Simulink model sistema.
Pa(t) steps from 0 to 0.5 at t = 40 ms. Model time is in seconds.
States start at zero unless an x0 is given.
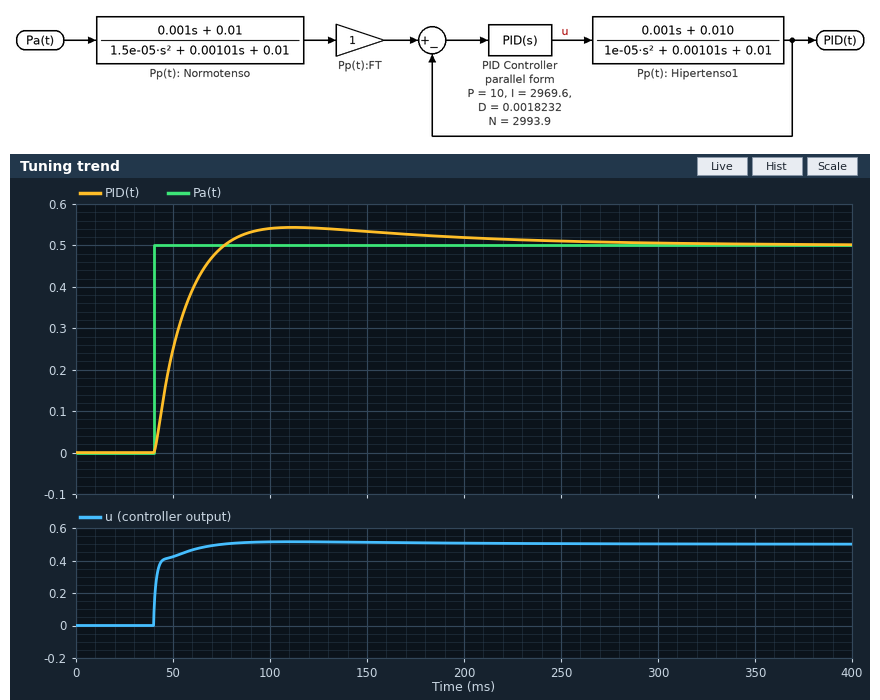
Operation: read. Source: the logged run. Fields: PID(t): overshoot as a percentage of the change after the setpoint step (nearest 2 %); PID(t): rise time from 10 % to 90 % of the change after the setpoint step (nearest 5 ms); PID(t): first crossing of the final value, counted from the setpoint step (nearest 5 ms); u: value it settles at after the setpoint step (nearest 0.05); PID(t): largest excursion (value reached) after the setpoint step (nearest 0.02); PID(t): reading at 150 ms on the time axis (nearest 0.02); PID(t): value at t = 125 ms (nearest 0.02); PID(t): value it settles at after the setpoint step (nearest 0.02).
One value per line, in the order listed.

8 %
25 ms
35 ms
0.50
0.54
0.54
0.54
0.50
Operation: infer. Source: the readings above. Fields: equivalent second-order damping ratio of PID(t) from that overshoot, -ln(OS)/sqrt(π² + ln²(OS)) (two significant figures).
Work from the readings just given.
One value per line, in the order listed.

0.63
